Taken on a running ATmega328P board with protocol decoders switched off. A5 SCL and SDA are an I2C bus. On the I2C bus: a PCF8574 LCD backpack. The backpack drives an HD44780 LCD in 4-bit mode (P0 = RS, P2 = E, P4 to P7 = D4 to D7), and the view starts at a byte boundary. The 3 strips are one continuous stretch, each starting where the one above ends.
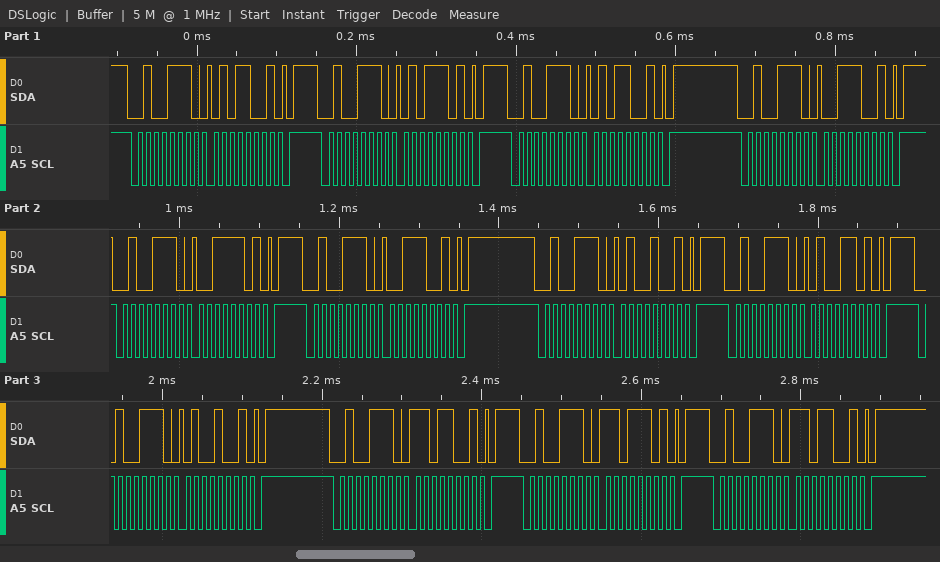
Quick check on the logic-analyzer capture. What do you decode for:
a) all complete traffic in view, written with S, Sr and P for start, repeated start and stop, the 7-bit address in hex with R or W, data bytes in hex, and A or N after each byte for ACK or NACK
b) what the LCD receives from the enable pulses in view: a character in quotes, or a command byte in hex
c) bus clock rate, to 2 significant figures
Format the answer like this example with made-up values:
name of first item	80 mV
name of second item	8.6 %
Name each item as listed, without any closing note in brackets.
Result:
all complete traffic in view, written with S, Sr and P for start, repeated start and stop, the 7-bit address in hex with R or W, data bytes in hex, and A or N after each byte for ACK or NACK	S 27W A 59 A P S 27W A 5D A P S 27W A 59 A P S 27W A 39 A P S 27W A 3D A P S 27W A 39 A P S 27W A 49 A P S 27W A 4D A P S 27W A 49 A P S 27W A D9 A P S 27W A DD A P S 27W A D9 A P
what the LCD receives from the enable pulses in view: a character in quotes, or a command byte in hex	'S' 'M'
bus clock rate, to 2 significant figures	100 kHz
